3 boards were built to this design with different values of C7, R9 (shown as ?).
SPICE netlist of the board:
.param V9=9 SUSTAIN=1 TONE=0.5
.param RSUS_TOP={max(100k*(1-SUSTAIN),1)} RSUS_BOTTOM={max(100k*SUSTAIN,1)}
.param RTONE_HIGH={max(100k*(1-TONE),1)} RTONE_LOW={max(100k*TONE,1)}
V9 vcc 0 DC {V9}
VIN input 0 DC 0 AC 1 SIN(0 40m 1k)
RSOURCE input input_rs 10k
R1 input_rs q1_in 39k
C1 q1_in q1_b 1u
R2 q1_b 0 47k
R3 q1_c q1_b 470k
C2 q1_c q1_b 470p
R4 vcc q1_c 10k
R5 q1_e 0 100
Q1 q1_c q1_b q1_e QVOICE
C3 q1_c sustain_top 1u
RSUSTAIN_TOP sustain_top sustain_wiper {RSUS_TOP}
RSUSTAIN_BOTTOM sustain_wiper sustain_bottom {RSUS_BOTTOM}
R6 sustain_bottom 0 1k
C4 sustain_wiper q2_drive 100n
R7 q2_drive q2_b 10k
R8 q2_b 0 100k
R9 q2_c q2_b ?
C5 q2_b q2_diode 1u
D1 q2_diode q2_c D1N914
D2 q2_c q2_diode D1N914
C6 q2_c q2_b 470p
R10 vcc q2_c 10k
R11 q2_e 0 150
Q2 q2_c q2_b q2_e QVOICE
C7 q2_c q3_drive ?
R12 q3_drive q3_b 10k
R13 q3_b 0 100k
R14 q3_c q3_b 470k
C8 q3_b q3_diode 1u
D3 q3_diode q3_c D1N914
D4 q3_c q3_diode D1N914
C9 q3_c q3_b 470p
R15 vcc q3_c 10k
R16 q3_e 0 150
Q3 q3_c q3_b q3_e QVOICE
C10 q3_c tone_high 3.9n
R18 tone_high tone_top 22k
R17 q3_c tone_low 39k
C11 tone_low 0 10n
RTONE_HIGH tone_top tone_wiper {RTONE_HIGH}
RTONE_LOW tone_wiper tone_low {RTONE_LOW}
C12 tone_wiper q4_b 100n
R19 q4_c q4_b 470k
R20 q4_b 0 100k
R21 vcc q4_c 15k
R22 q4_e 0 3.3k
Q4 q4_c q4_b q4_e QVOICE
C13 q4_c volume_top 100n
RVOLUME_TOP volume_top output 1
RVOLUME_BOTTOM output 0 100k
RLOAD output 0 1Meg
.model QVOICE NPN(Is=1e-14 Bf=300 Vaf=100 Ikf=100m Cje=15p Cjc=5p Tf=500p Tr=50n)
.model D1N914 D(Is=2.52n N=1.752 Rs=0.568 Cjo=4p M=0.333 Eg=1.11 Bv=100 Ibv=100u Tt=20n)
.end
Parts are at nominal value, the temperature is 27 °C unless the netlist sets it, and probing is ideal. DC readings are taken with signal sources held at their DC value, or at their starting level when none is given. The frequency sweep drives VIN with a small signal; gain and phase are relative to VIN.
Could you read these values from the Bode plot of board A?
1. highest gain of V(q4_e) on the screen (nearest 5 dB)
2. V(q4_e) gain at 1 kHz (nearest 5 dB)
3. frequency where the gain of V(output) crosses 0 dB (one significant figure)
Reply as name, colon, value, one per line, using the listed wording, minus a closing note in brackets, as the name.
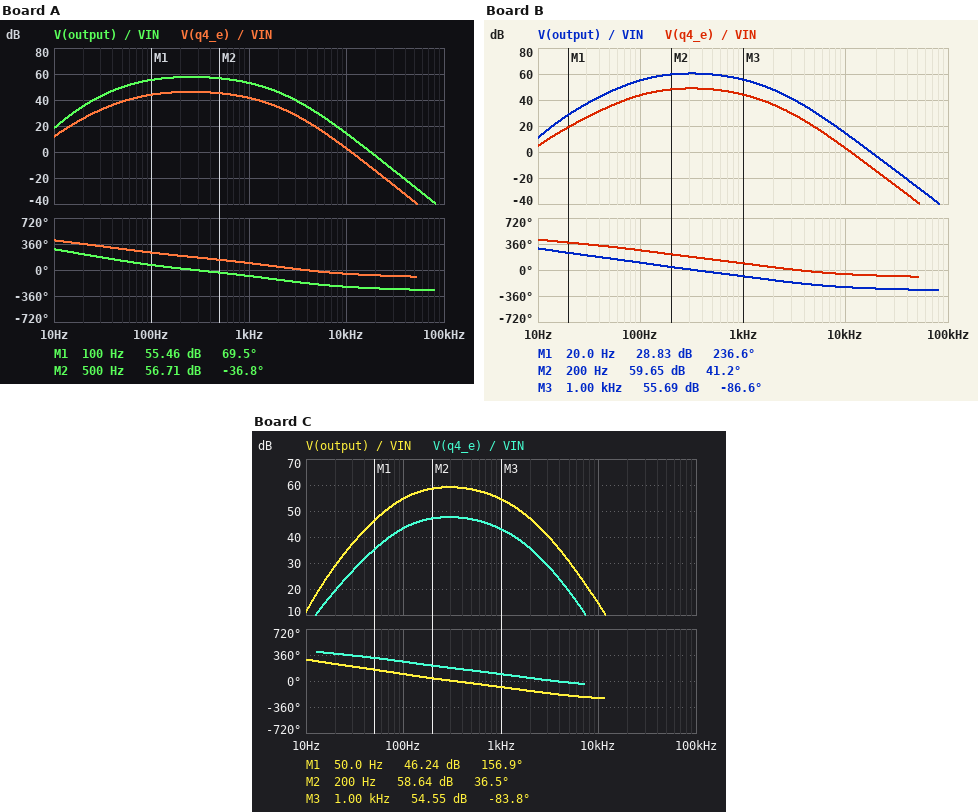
highest gain of V(q4_e) on the screen: 45 dB
V(q4_e) gain at 1 kHz: 40 dB
frequency where the gain of V(output) crosses 0 dB: 20 kHz
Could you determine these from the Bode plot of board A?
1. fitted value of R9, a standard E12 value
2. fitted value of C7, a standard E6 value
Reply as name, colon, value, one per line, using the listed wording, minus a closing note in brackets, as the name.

fitted value of R9, a standard E12 value: 150 kΩ
fitted value of C7, a standard E6 value: 220 nF
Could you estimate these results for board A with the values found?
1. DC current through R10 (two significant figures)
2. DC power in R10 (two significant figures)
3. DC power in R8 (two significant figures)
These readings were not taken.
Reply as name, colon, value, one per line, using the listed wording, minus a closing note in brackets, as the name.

DC current through R10: 680 µA
DC power in R10: 4.6 mW
DC power in R8: 5.6 µW
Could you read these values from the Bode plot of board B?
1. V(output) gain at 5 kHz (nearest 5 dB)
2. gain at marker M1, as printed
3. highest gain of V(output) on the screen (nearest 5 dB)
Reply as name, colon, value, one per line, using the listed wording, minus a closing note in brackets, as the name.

V(output) gain at 5 kHz: 30 dB
gain at marker M1, as printed: 28.83 dB
highest gain of V(output) on the screen: 60 dB
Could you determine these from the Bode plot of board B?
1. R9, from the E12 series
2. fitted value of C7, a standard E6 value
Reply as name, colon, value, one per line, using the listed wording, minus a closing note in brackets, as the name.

R9, from the E12 series: 330 kΩ
fitted value of C7, a standard E6 value: 47 nF
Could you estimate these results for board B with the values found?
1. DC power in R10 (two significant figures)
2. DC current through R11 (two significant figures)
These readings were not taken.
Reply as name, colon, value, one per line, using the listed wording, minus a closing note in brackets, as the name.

DC power in R10: 2.9 mW
DC current through R11: 530 µA
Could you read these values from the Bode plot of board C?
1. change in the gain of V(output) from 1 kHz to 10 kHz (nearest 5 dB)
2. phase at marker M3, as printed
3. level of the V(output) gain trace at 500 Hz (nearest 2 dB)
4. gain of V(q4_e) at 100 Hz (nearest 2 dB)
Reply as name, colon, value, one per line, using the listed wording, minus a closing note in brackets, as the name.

change in the gain of V(output) from 1 kHz to 10 kHz: -40 dB
phase at marker M3, as printed: -83.8 deg
level of the V(output) gain trace at 500 Hz: 58 dB
gain of V(q4_e) at 100 Hz: 44 dB
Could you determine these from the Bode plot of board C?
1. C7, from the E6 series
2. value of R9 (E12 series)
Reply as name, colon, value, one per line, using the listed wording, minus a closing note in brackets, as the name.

C7, from the E6 series: 68 nF
value of R9: 220 kΩ
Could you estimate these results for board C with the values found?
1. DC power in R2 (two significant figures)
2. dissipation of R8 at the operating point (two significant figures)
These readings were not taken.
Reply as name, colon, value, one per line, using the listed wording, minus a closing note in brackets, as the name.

DC power in R2: 8.3 µW
dissipation of R8 at the operating point: 5.4 µW
